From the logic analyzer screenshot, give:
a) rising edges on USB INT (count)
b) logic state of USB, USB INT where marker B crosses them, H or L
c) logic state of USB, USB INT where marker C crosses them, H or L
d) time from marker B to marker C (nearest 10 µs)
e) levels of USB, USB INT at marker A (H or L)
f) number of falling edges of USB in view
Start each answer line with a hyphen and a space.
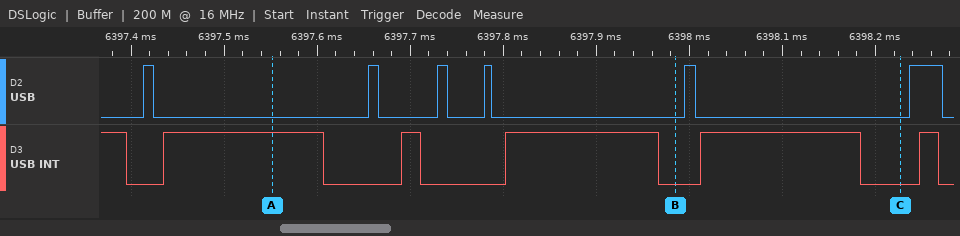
- 5
- USB=L, USB INT=L
- USB=L, USB INT=L
- 240 µs
- USB=L, USB INT=H
- 6
